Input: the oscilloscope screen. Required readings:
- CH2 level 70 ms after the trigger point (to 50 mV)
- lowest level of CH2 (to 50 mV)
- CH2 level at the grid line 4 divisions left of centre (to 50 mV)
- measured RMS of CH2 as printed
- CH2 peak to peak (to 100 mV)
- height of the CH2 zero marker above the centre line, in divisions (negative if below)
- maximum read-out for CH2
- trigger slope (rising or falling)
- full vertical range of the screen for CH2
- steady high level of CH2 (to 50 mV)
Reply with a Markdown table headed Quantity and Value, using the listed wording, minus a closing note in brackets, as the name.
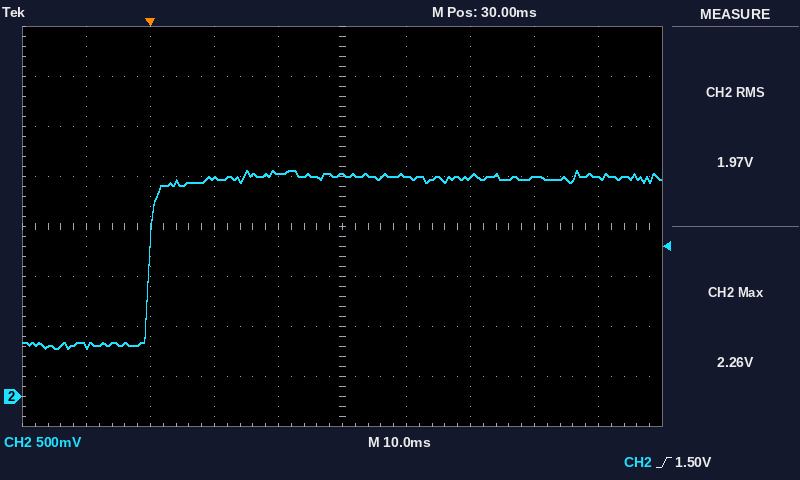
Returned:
| Quantity | Value |
|---|---|
| CH2 level 70 ms after the trigger point | 2.20 V |
| lowest level of CH2 | 500 mV |
| CH2 level at the grid line 4 divisions left of centre | 500 mV |
| measured RMS of CH2 as printed | 1.97 V |
| CH2 peak to peak | 1.80 V |
| height of the CH2 zero marker above the centre line, in divisions | -3.4 div |
| maximum read-out for CH2 | 2.26 V |
| trigger slope | rising |
| full vertical range of the screen for CH2 | 4 V |
| steady high level of CH2 | 2.20 V |
